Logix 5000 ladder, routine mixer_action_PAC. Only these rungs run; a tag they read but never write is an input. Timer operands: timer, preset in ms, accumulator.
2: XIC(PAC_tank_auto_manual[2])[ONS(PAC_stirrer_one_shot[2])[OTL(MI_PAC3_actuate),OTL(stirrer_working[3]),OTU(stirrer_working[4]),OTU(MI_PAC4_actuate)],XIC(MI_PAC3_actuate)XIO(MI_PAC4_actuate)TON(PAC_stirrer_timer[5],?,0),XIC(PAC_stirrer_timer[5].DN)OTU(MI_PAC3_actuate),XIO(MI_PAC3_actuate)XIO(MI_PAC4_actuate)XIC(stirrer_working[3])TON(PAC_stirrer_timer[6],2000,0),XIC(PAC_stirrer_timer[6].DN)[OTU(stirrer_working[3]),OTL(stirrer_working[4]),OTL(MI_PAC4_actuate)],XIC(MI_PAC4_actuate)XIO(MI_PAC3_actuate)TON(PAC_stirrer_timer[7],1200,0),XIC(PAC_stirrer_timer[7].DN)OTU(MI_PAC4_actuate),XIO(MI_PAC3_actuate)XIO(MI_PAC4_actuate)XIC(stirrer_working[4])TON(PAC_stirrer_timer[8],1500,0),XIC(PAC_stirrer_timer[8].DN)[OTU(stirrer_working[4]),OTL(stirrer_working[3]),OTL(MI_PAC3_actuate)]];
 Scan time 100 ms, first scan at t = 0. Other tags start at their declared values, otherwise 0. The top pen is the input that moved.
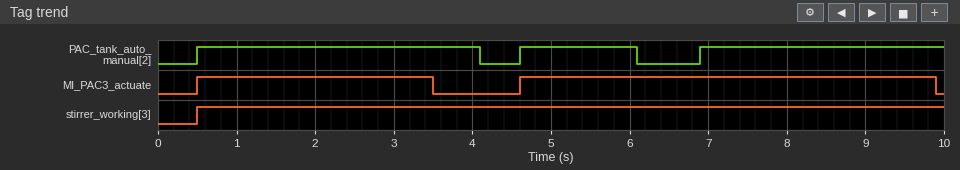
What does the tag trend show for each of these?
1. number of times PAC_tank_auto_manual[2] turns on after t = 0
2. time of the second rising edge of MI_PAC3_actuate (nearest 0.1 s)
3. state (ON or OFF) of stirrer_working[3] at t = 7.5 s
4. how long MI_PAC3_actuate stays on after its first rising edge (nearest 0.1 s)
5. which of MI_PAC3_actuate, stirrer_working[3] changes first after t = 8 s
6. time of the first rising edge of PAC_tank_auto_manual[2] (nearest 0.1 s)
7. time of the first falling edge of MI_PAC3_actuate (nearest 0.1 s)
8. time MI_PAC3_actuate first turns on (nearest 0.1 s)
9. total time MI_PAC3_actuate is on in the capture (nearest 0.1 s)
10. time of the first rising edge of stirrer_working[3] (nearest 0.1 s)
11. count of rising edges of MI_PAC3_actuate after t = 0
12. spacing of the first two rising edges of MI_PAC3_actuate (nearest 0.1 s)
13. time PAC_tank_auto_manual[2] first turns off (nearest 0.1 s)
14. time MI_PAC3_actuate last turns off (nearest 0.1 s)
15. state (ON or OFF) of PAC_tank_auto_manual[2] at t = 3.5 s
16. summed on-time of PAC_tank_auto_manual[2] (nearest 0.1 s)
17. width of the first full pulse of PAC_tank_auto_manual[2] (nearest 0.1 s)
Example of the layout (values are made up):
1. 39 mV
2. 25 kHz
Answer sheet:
1. 3
2. 4.6 s
3. ON
4. 3.0 s
5. MI_PAC3_actuate
6. 0.5 s
7. 3.5 s
8. 0.5 s
9. 8.3 s
10. 0.5 s
11. 2
12. 4.1 s
13. 4.1 s
14. 9.9 s
15. ON
16. 8.2 s
17. 3.6 s
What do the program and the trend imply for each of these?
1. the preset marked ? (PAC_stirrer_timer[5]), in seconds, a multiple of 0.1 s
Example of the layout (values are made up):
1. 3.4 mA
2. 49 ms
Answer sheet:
1. 3.0 s
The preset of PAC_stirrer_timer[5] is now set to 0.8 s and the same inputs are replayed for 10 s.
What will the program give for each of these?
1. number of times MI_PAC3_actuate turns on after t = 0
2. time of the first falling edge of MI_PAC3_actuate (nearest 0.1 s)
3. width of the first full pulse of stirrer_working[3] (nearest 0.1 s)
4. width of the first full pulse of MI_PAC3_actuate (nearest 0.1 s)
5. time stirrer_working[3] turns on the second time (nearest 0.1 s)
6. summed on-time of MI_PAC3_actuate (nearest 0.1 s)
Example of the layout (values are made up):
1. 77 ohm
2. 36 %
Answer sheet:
1. 3
2. 1.3 s
3. 2.8 s
4. 0.8 s
5. 4.6 s
6. 2.4 s
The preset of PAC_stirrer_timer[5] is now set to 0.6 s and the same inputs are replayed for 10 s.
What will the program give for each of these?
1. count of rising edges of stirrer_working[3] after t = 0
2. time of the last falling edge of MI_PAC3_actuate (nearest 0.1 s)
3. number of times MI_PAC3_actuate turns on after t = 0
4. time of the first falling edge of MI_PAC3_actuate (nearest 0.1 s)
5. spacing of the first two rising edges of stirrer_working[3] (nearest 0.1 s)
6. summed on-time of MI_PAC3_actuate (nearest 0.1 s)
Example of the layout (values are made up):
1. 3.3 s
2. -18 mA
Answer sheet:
1. 2
2. 7.5 s
3. 3
4. 1.1 s
5. 4.1 s
6. 1.8 s
